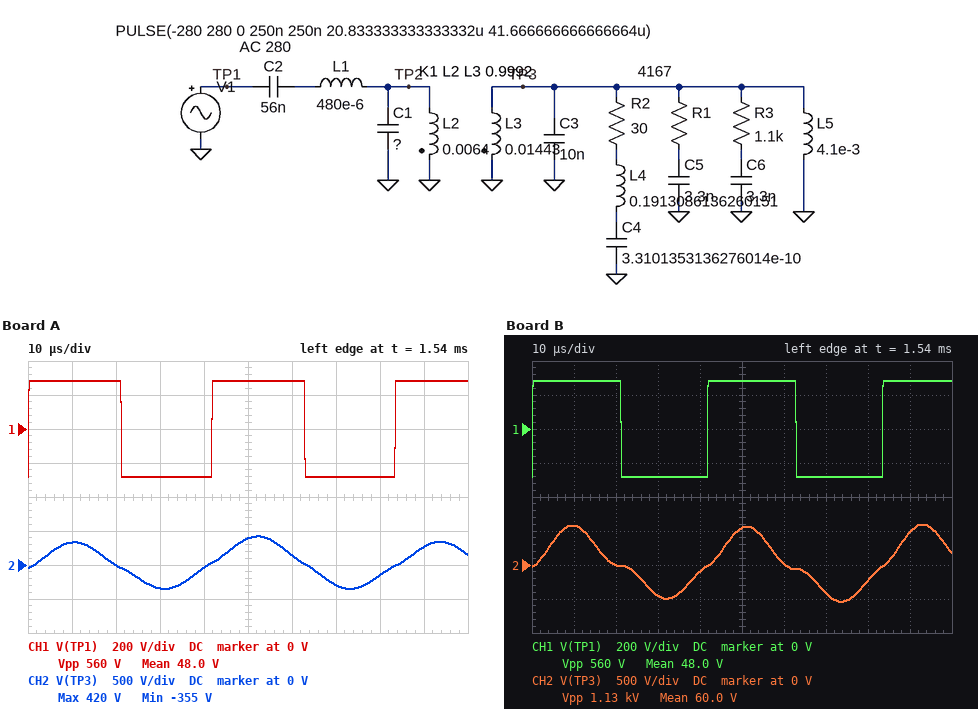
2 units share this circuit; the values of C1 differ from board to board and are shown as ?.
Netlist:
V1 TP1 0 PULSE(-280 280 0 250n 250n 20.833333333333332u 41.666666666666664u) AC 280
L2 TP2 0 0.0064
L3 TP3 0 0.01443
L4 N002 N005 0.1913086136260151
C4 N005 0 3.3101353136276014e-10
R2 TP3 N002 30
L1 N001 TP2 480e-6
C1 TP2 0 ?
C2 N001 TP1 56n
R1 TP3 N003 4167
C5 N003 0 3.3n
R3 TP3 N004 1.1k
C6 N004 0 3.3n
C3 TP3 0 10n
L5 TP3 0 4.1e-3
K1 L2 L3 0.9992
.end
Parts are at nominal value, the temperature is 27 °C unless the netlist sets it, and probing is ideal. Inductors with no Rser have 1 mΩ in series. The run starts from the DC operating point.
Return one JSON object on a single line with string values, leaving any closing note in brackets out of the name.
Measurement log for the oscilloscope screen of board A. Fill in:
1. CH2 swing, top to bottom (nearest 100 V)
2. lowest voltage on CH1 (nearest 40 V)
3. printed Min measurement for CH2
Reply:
{"CH2 swing, top to bottom": "800 V", "lowest voltage on CH1": "-280 V", "printed Min measurement for CH2": "-355 V"}
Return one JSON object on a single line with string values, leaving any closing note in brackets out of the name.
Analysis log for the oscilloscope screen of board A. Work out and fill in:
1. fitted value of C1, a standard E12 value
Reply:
{"fitted value of C1, a standard E12 value": "82 nF"}
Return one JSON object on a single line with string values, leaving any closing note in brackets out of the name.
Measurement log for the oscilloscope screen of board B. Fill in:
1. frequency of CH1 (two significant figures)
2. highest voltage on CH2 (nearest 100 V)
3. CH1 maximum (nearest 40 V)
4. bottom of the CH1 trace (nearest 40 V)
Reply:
{"frequency of CH1": "24 kHz", "highest voltage on CH2": "600 V", "CH1 maximum": "280 V", "bottom of the CH1 trace": "-280 V"}
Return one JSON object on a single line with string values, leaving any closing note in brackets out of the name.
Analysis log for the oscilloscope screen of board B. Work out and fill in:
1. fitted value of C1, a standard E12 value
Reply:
{"fitted value of C1, a standard E12 value": "22 nF"}
